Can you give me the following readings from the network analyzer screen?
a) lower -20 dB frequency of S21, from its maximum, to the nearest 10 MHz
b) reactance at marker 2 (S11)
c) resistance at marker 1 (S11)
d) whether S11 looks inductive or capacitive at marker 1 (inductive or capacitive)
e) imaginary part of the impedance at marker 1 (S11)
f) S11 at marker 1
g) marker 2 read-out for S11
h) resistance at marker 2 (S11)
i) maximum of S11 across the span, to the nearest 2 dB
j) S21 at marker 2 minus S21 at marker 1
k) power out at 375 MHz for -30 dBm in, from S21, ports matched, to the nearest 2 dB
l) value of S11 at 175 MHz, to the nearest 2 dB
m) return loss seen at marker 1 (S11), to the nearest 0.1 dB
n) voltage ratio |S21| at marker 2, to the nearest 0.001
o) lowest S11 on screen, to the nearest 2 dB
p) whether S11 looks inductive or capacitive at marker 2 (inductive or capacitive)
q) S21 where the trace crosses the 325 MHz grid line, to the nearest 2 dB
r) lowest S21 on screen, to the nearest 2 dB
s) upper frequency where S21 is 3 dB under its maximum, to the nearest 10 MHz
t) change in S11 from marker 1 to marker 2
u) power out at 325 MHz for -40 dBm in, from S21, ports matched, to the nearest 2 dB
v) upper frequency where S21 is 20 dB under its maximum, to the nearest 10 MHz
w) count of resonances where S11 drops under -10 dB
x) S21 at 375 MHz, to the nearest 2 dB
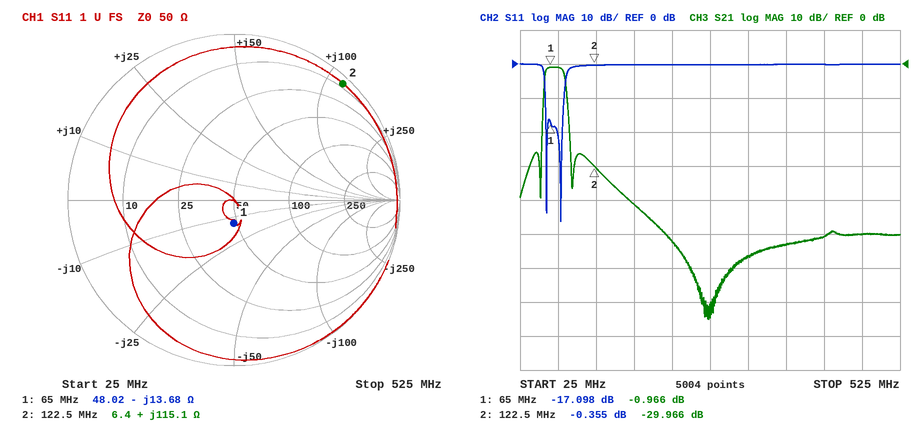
50 MHz
+115.1 Ω
48.02 Ω
capacitive
-13.68 Ω
-17.098 dB
-0.355 dB
6.4 Ω
0 dB
-29.000 dB
-84 dBm
0 dB
17.1 dB
0.032
-46 dB
inductive
-56 dB
-76 dB
80 MHz
16.743 dB
-96 dBm
90 MHz
2
-54 dB
